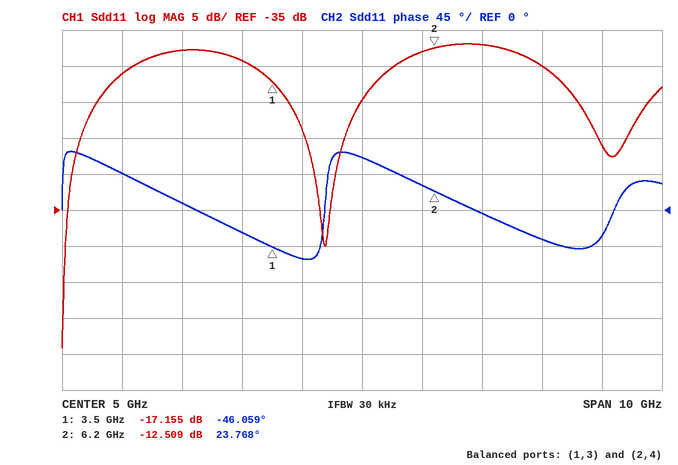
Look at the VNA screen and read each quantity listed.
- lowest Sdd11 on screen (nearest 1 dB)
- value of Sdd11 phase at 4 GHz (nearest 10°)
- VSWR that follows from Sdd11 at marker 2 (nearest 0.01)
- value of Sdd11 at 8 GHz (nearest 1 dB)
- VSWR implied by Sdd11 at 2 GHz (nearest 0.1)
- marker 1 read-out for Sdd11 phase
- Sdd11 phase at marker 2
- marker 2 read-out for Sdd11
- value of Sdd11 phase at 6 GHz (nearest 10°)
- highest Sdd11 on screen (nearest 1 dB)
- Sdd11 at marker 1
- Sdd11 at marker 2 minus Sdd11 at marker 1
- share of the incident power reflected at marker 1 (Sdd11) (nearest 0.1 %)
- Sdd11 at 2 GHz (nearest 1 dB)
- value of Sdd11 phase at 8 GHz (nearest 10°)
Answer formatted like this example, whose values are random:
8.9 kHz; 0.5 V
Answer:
-54 dB; -60°; 1.62; -15 dB; 1.6; -46.059°; 23.768°; -12.509 dB; 30°; -12 dB; -17.155 dB; 4.646 dB; 1.9 %; -13 dB; -40°
